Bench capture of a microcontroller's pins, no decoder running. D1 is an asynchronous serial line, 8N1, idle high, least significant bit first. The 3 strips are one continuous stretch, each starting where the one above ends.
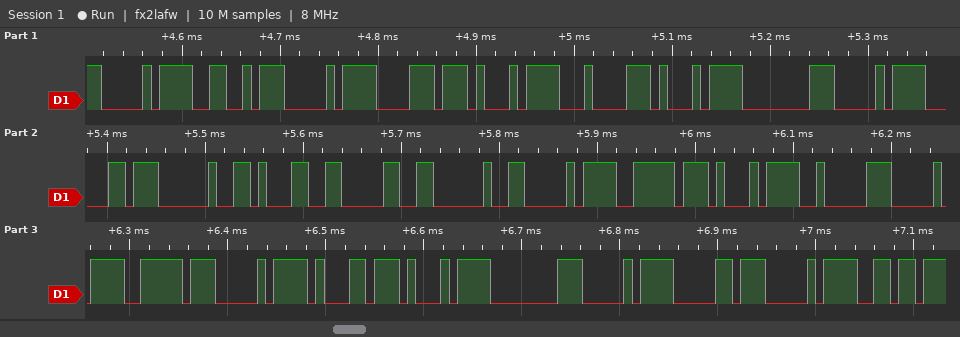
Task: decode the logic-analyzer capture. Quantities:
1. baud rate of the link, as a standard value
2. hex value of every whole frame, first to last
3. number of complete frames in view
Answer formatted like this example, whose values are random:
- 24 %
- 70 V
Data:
- 115200 baud
- D0 A6 D0 B8 D1 84 D1 80 D0 B0 20 31 30 20 D0 BE D1 82 D0 BE D0 B1 D1 80 D0 B0 D0 B6
- 28
